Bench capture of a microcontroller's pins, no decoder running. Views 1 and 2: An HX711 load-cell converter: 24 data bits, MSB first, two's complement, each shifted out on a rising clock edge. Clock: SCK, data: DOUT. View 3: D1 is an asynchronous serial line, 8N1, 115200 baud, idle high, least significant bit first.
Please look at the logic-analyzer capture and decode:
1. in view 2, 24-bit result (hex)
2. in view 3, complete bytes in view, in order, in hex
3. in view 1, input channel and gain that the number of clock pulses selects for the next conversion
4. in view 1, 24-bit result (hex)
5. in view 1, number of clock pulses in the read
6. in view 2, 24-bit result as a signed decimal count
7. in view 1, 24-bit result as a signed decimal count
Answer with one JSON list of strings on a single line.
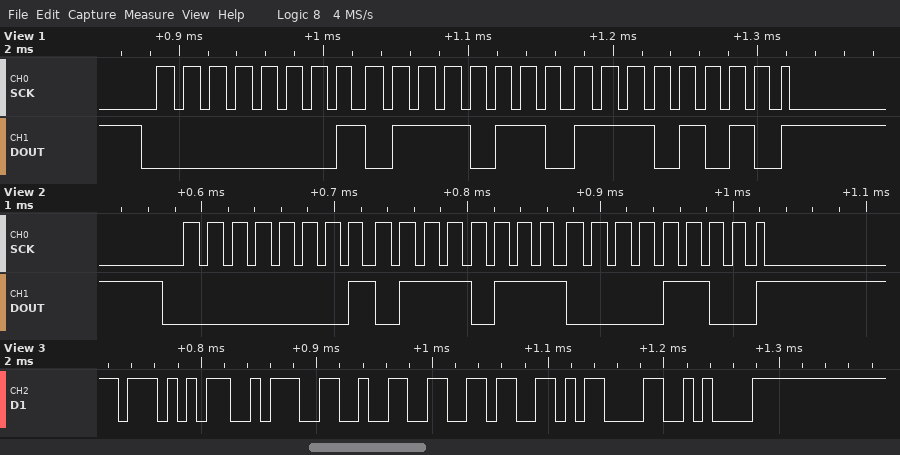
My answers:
["0x01770C", "0x57 0x3A 0x32 0x36 0x0D 0x0A", "channel A, gain 128", "0x0176EA", "25", "96012", "95978"]
